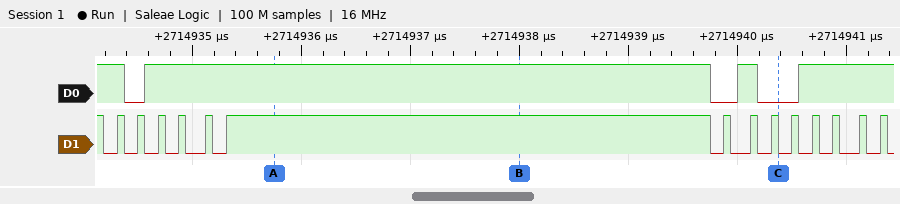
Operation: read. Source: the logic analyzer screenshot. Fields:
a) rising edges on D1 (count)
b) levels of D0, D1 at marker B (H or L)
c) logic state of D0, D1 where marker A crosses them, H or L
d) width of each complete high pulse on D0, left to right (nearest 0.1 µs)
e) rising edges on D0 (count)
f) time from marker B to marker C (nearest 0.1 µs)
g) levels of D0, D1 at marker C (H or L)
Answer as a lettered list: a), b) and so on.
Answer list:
a) 14
b) D0=H, D1=H
c) D0=H, D1=H
d) 5.2 µs, 0.2 µs
e) 3
f) 2.4 µs
g) D0=L, D1=L
